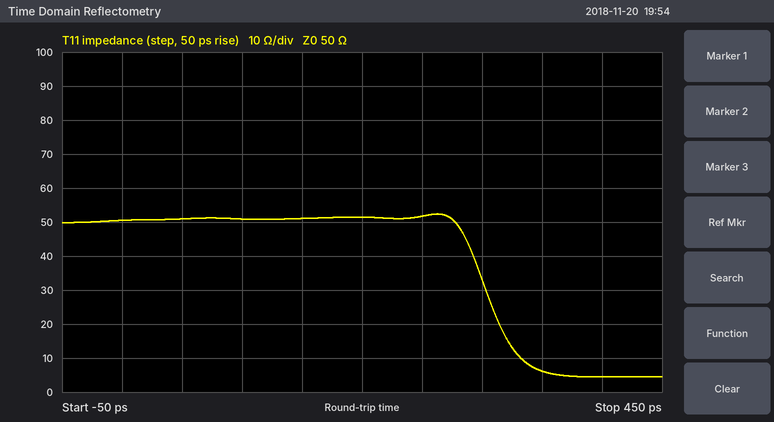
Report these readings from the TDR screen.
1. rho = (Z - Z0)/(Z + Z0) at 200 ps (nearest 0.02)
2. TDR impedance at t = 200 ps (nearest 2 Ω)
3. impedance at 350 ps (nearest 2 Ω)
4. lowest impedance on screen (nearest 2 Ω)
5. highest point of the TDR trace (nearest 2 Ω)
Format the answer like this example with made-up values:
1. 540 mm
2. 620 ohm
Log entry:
1. +0.02
2. 52 Ω
3. 6 Ω
4. 4 Ω
5. 52 Ω
